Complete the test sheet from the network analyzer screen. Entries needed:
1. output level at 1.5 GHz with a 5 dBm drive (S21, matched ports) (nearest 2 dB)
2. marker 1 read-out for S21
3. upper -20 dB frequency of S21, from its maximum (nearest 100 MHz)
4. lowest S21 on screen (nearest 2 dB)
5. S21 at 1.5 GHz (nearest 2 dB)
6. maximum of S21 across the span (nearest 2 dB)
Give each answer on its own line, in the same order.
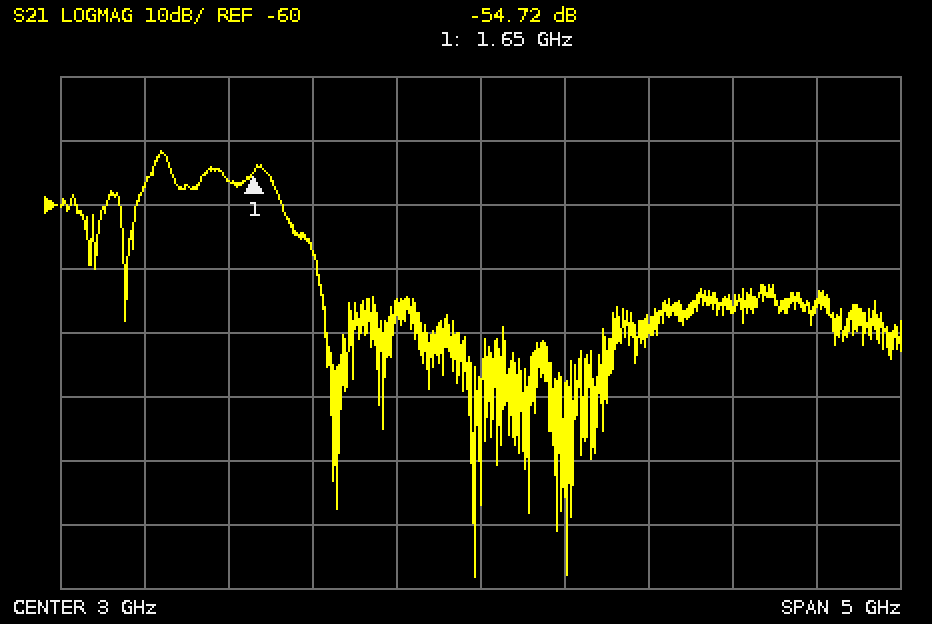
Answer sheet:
-52 dBm
-54.72 dB
2.0 GHz
-118 dB
-56 dB
-52 dB
